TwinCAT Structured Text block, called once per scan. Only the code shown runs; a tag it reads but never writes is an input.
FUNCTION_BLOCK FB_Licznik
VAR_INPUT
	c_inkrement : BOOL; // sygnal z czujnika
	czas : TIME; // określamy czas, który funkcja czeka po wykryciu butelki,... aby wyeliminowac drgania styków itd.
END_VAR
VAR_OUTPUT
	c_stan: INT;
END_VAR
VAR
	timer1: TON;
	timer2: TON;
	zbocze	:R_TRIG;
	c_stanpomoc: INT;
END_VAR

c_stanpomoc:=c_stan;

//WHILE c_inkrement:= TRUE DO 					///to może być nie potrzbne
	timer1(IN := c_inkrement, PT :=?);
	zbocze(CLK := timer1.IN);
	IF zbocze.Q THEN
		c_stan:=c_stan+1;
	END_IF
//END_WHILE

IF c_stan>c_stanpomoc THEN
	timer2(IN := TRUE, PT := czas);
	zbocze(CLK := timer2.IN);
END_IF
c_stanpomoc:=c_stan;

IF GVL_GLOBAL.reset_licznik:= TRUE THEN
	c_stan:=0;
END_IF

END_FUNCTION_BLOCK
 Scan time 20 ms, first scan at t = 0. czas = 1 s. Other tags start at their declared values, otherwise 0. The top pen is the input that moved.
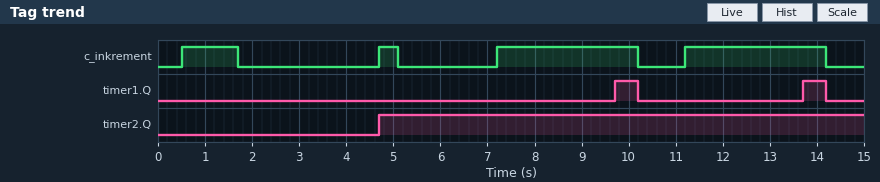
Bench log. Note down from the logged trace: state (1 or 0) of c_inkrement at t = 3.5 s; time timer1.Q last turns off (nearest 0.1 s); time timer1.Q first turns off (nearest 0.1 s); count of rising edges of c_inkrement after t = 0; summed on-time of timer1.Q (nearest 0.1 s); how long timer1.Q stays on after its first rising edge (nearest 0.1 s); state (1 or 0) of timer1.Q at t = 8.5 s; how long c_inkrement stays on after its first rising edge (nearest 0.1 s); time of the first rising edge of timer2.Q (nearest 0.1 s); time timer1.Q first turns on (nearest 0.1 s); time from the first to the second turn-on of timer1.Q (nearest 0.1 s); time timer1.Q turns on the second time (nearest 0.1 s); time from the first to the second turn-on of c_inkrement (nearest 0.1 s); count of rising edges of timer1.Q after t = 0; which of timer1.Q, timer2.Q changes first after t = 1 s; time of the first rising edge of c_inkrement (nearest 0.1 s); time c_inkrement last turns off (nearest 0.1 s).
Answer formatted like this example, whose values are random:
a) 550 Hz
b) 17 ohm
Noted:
a) 0
b) 14.2 s
c) 10.2 s
d) 4
e) 1.0 s
f) 0.5 s
g) 0
h) 1.2 s
i) 4.7 s
j) 9.7 s
k) 4.0 s
l) 13.7 s
m) 4.2 s
n) 2
o) timer2.Q
p) 0.5 s
q) 14.2 s
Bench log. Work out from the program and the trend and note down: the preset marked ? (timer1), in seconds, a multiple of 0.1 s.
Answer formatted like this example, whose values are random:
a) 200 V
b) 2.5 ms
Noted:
a) 2.5 s
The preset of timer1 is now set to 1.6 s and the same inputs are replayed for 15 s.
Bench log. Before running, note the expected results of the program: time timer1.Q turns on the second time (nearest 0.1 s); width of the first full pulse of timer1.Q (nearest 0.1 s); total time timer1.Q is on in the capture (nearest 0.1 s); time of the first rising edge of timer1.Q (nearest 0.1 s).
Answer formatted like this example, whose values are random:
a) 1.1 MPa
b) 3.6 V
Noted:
a) 12.8 s
b) 1.4 s
c) 2.8 s
d) 8.8 s
